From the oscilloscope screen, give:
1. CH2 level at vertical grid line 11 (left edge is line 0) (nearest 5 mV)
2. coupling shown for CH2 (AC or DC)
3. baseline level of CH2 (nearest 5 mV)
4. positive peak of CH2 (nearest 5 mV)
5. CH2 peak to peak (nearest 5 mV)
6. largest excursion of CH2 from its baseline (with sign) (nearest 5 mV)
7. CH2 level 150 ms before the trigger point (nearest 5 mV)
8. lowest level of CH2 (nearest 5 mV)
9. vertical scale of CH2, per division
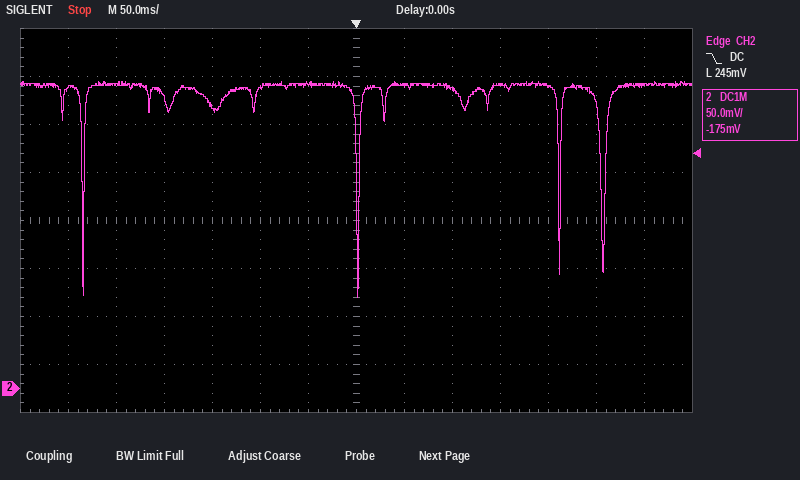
315 mV
DC
315 mV
320 mV
225 mV
-220 mV
295 mV
95 mV
50 mV
